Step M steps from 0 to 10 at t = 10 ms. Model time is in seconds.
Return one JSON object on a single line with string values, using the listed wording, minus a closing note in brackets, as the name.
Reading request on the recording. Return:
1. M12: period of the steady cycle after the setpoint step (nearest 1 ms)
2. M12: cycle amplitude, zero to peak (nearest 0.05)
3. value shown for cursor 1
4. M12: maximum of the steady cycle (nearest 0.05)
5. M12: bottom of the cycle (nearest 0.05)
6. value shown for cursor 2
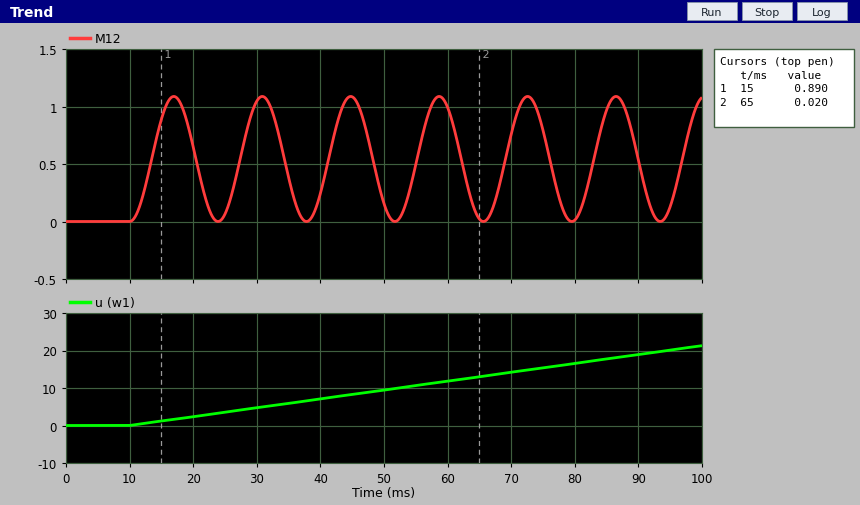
{"M12: period of the steady cycle after the setpoint step": "14 ms", "M12: cycle amplitude, zero to peak": "0.55", "value shown for cursor 1": "0.890", "M12: maximum of the steady cycle": "1.10", "M12: bottom of the cycle": "0.00", "value shown for cursor 2": "0.020"}
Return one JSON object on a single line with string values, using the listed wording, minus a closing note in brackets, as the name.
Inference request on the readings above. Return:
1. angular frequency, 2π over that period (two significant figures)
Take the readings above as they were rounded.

{"angular frequency, 2π over that period": "0.45 rad/ms"}
